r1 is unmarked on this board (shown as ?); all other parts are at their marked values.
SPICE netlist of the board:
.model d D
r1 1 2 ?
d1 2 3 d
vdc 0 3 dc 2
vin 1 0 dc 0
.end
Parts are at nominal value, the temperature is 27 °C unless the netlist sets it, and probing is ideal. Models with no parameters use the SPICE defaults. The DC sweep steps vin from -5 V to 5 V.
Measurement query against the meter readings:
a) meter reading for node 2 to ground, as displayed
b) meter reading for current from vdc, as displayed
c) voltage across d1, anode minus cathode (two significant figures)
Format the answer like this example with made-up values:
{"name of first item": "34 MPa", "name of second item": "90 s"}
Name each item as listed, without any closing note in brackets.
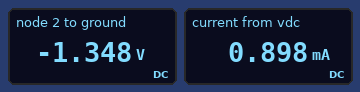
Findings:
{"meter reading for node 2 to ground, as displayed": "-1.348 V", "meter reading for current from vdc, as displayed": "0.898 mA", "voltage across d1, anode minus cathode": "650 mV"}
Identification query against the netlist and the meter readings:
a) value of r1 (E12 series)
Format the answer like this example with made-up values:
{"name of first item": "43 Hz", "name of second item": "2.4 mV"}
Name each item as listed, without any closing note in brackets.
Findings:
{"value of r1": "1.5 kΩ"}
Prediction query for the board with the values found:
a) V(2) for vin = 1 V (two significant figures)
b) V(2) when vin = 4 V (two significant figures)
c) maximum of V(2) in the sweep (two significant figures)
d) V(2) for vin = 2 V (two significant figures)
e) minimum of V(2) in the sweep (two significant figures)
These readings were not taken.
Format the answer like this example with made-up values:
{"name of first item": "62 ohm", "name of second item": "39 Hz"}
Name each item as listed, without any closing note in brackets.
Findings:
{"V(2) for vin = 1 V": "-1.3 V", "V(2) when vin = 4 V": "-1.3 V", "maximum of V(2) in the sweep": "-1.3 V", "V(2) for vin = 2 V": "-1.3 V", "minimum of V(2) in the sweep": "-5.0 V"}
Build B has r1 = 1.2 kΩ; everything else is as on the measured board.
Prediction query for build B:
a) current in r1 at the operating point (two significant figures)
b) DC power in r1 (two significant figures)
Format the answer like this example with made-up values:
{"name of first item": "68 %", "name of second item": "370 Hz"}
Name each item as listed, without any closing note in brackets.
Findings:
{"current in r1 at the operating point": "1.1 mA", "DC power in r1": "1.5 mW"}
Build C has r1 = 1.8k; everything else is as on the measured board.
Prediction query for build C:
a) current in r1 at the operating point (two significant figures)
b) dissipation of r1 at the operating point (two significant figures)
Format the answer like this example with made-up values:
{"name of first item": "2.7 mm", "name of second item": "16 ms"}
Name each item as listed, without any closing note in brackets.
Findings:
{"current in r1 at the operating point": "750 µA", "dissipation of r1 at the operating point": "1.0 mW"}
